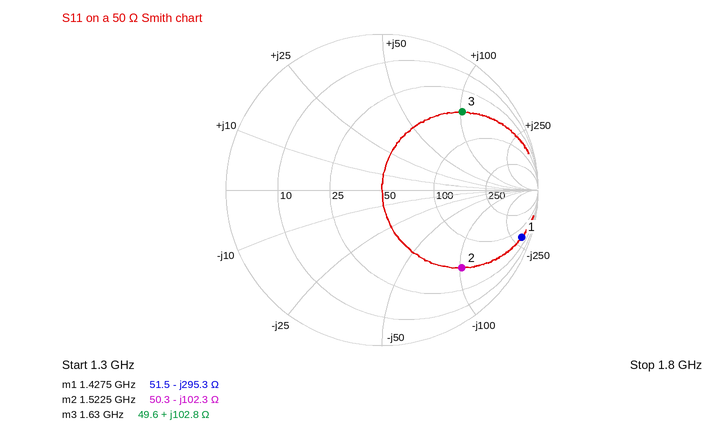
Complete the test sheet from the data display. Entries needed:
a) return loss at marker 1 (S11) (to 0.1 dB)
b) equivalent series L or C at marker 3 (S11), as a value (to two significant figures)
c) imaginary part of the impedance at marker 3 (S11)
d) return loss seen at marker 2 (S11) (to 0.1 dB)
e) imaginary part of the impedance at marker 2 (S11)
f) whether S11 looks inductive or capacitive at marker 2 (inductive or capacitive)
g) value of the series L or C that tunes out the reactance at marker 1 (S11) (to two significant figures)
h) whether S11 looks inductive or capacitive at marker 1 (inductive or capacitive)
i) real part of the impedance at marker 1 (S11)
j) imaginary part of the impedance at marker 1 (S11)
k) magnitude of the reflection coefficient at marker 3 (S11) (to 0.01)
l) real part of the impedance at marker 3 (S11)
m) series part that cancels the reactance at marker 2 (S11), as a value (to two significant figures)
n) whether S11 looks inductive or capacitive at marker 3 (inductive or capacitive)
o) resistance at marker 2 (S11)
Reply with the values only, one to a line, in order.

0.5 dB
10 nH
+102.8 Ω
2.9 dB
-102.3 Ω
capacitive
33 nH
capacitive
51.5 Ω
-295.3 Ω
0.72
49.6 Ω
11 nH
inductive
50.3 Ω
